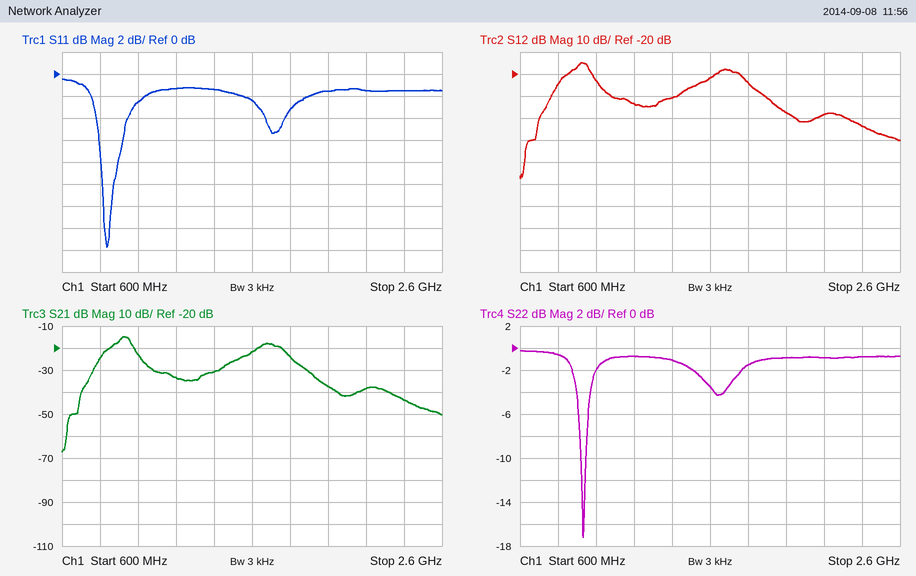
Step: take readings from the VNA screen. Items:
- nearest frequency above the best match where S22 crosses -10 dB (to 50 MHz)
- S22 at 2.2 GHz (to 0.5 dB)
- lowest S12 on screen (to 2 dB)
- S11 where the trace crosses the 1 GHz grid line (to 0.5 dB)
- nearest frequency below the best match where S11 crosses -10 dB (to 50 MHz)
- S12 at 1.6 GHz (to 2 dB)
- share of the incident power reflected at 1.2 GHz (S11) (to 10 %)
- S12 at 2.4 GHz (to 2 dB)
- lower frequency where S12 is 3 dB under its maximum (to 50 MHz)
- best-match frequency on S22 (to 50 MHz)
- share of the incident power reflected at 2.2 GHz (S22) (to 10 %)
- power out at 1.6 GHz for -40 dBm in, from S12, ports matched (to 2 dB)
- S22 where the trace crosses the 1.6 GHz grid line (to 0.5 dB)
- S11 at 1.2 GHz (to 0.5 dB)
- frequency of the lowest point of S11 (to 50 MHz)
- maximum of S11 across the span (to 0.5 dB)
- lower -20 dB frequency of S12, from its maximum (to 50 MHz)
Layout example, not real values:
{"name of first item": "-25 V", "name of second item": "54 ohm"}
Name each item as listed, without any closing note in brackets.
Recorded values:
{"nearest frequency above the best match where S22 crosses -10 dB": "950 MHz", "S22 at 2.2 GHz": "-1.0 dB", "lowest S12 on screen": "-68 dB", "S11 where the trace crosses the 1 GHz grid line": "-2.5 dB", "nearest frequency below the best match where S11 crosses -10 dB": "800 MHz", "S12 at 1.6 GHz": "-22 dB", "share of the incident power reflected at 1.2 GHz (S11)": "70 %", "S12 at 2.4 GHz": "-44 dB", "lower frequency where S12 is 3 dB under its maximum": "900 MHz", "best-match frequency on S22": "950 MHz", "share of the incident power reflected at 2.2 GHz (S22)": "80 %", "power out at 1.6 GHz for -40 dBm in, from S12, ports matched": "-62 dBm", "S22 where the trace crosses the 1.6 GHz grid line": "-3.5 dB", "S11 at 1.2 GHz": "-1.5 dB", "frequency of the lowest point of S11": "850 MHz", "maximum of S11 across the span": "-0.5 dB", "lower -20 dB frequency of S12, from its maximum": "750 MHz"}
